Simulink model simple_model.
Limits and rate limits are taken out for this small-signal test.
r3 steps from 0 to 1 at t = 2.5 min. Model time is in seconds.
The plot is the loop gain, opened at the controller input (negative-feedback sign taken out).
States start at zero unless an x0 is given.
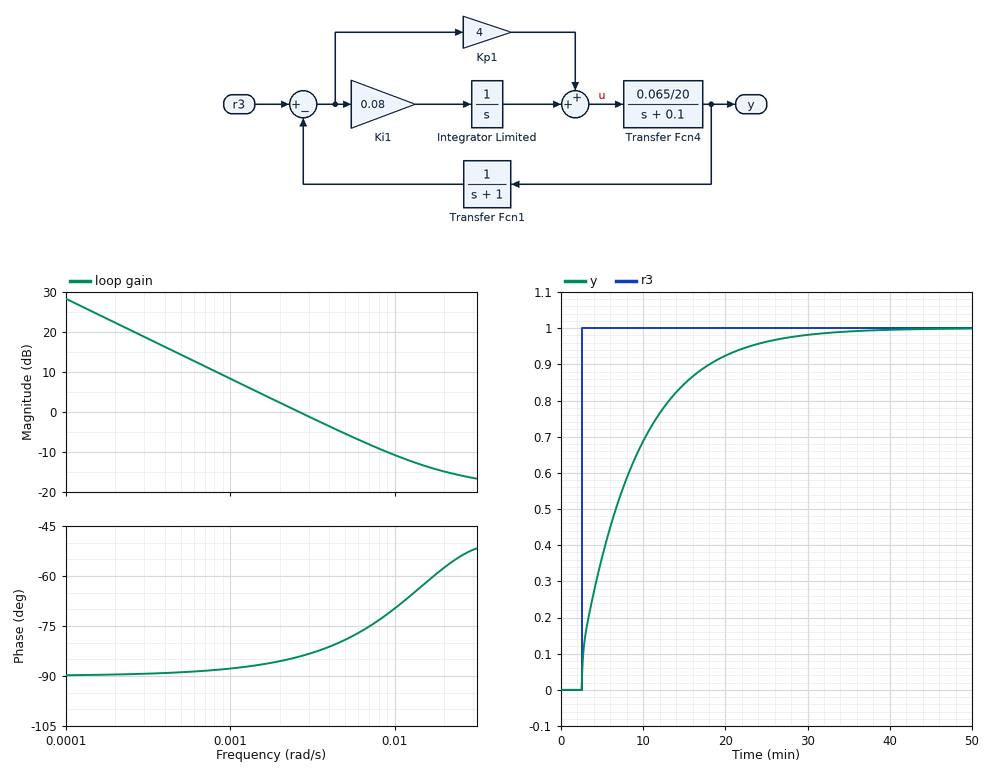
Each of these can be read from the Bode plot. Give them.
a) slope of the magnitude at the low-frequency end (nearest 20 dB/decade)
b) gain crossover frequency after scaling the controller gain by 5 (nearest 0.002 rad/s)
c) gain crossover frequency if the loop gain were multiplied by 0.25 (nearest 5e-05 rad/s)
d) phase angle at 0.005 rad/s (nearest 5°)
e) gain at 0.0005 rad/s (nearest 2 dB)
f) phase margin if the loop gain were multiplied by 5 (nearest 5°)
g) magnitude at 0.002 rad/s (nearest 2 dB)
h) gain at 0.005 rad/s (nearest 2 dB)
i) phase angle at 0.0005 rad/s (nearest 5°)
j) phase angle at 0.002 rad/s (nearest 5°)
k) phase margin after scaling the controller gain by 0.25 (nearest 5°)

-20 dB/decade
0.016 rad/s
0.00065 rad/s
-80°
14 dB
120°
2 dB
-6 dB
-90°
-85°
90°
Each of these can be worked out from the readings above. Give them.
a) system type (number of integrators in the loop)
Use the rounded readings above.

1
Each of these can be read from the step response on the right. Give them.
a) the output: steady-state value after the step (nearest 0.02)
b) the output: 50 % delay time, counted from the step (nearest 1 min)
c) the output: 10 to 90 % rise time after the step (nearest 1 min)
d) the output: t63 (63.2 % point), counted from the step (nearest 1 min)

1.00
4 min
15 min
6 min
